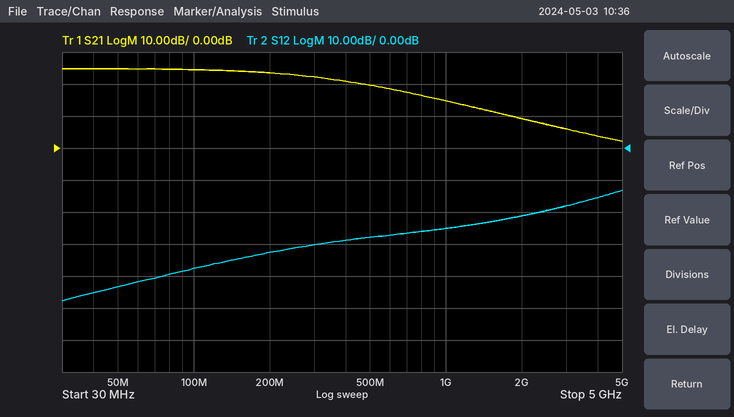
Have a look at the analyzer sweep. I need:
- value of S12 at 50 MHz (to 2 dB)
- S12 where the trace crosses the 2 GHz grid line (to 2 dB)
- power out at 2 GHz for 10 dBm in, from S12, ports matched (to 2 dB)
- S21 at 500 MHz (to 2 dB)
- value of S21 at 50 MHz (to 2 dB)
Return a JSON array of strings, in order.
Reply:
["-44 dB", "-22 dB", "-12 dBm", "20 dB", "24 dB"]
